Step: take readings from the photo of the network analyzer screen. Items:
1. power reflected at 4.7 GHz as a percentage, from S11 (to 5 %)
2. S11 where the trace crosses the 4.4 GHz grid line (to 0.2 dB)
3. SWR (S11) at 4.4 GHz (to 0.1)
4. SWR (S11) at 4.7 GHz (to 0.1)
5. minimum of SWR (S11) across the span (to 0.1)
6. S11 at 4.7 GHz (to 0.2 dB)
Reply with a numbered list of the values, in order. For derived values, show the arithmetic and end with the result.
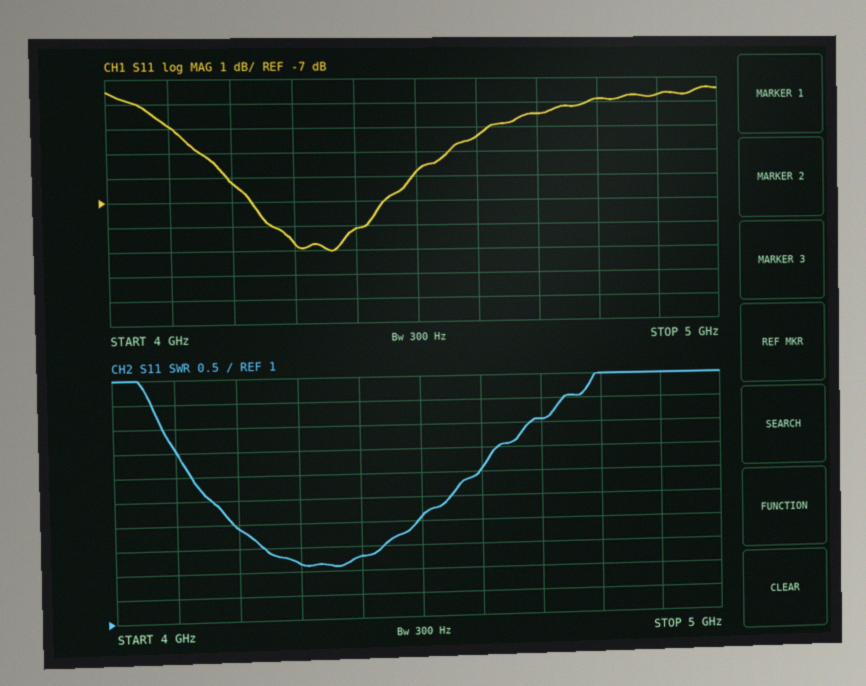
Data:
1. 10^(-3.4/10) ≈ 45.7 %, so 45 % to the nearest 5 %
2. -8.2 dB
3. 2.3
4. 5.1
5. 2.1
6. -3.4 dB
